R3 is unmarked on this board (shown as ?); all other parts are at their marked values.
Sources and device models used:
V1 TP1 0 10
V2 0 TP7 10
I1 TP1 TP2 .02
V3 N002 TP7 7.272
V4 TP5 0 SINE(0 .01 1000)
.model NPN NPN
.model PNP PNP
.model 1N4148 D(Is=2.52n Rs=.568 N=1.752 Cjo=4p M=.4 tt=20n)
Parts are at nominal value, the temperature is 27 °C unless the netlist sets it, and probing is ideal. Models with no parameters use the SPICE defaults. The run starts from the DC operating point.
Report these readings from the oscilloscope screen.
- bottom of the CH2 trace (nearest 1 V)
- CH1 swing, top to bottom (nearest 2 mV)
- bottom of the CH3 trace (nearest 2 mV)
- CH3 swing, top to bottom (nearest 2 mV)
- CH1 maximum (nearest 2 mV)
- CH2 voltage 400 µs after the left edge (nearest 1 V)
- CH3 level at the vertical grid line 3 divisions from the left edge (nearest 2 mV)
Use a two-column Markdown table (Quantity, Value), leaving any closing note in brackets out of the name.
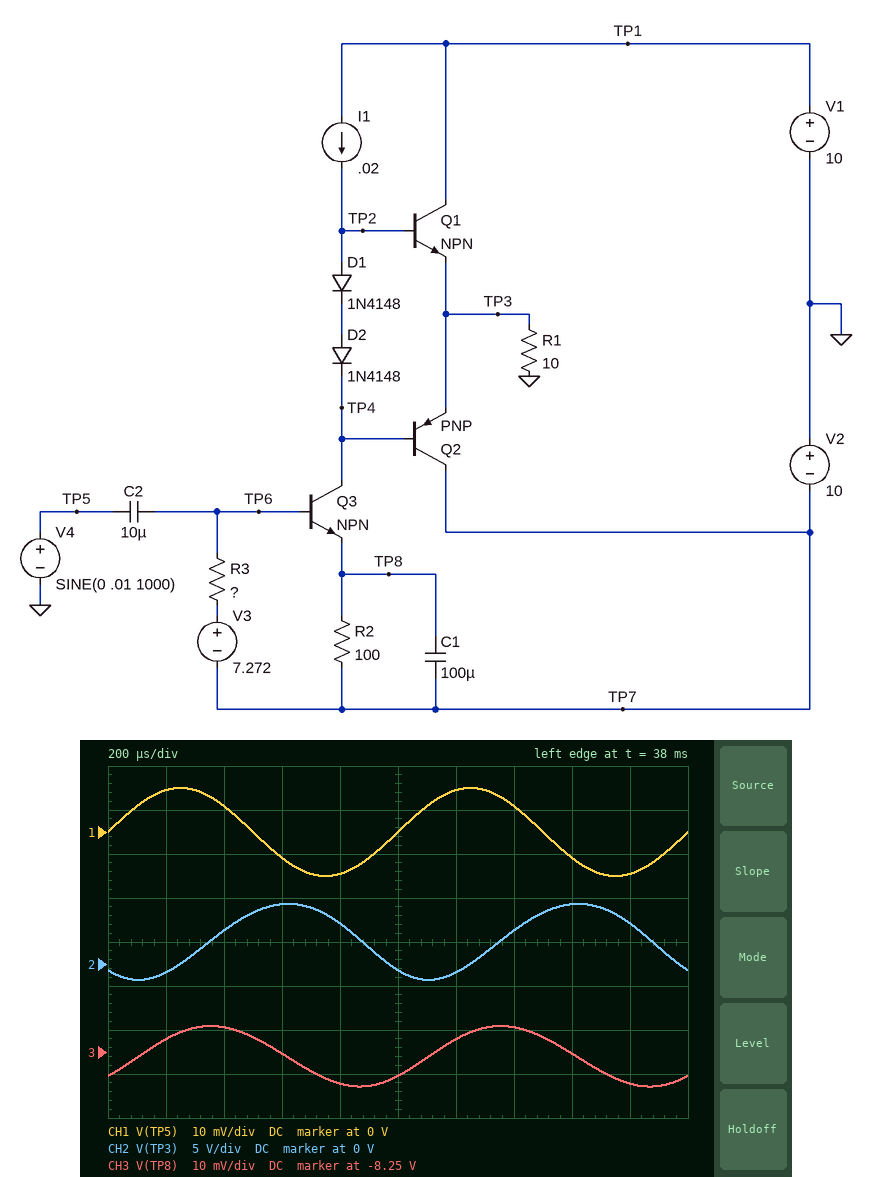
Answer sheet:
| Quantity | Value |
|---|---|
| bottom of the CH2 trace | -2 V |
| CH1 swing, top to bottom | 20 mV |
| bottom of the CH3 trace | -8.258 V |
| CH3 swing, top to bottom | 14 mV |
| CH1 maximum | 10 mV |
| CH2 voltage 400 µs after the left edge | 4 V |
| CH3 level at the vertical grid line 3 divisions from the left edge | -8.250 V |
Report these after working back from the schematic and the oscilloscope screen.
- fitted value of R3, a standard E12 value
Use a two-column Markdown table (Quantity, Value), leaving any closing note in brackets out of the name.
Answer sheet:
| Quantity | Value |
|---|---|
| fitted value of R3, a standard E12 value | 27 kΩ |
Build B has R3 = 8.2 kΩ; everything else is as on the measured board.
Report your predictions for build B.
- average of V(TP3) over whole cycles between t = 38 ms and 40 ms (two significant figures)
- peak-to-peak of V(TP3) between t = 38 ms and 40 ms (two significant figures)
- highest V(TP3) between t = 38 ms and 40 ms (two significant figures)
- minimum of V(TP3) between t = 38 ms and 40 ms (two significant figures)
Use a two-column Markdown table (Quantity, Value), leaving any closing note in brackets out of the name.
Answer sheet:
| Quantity | Value |
|---|---|
| average of V(TP3) over whole cycles between t = 38 ms and 40 ms | -5.2 V |
| peak-to-peak of V(TP3) between t = 38 ms and 40 ms | 4.0 V |
| highest V(TP3) between t = 38 ms and 40 ms | -2.4 V |
| minimum of V(TP3) between t = 38 ms and 40 ms | -6.4 V |
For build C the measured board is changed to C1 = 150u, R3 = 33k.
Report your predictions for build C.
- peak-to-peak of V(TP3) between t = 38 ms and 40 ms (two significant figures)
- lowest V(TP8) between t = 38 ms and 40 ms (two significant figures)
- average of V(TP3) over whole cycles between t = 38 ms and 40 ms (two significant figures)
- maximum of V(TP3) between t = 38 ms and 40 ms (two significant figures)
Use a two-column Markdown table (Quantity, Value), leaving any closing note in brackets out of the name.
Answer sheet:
| Quantity | Value |
|---|---|
| peak-to-peak of V(TP3) between t = 38 ms and 40 ms | 9.4 V |
| lowest V(TP8) between t = 38 ms and 40 ms | -8.5 V |
| average of V(TP3) over whole cycles between t = 38 ms and 40 ms | 5.1 V |
| maximum of V(TP3) between t = 38 ms and 40 ms | 9.5 V |
